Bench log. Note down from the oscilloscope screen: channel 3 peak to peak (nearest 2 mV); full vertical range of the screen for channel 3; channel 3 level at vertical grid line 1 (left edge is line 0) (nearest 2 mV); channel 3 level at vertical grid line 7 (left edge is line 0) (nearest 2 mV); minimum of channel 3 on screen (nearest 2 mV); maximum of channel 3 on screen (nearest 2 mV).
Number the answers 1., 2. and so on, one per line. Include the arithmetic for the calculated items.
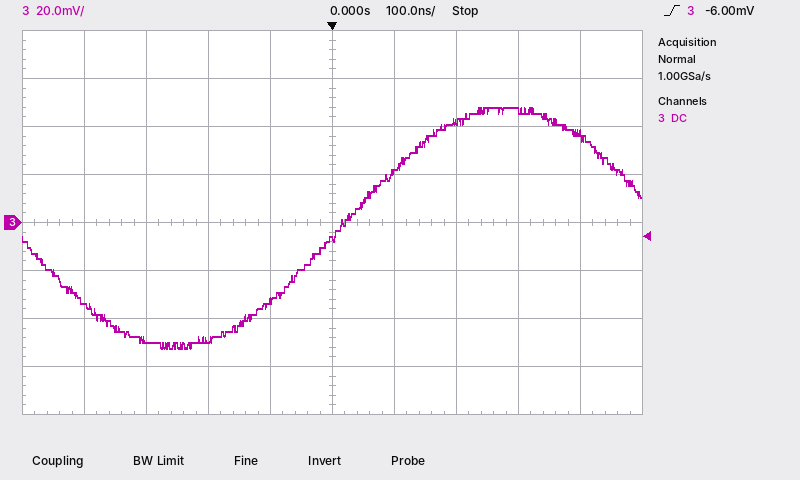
1. 48 mV − (-52 mV) = 100 mV
2. 160 mV
3. -34 mV
4. 42 mV
5. -52 mV
6. 48 mV
